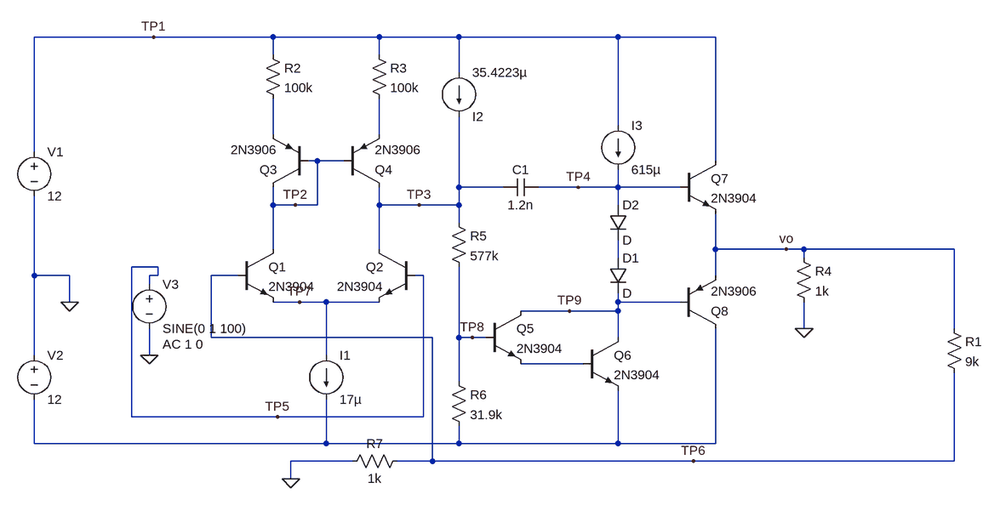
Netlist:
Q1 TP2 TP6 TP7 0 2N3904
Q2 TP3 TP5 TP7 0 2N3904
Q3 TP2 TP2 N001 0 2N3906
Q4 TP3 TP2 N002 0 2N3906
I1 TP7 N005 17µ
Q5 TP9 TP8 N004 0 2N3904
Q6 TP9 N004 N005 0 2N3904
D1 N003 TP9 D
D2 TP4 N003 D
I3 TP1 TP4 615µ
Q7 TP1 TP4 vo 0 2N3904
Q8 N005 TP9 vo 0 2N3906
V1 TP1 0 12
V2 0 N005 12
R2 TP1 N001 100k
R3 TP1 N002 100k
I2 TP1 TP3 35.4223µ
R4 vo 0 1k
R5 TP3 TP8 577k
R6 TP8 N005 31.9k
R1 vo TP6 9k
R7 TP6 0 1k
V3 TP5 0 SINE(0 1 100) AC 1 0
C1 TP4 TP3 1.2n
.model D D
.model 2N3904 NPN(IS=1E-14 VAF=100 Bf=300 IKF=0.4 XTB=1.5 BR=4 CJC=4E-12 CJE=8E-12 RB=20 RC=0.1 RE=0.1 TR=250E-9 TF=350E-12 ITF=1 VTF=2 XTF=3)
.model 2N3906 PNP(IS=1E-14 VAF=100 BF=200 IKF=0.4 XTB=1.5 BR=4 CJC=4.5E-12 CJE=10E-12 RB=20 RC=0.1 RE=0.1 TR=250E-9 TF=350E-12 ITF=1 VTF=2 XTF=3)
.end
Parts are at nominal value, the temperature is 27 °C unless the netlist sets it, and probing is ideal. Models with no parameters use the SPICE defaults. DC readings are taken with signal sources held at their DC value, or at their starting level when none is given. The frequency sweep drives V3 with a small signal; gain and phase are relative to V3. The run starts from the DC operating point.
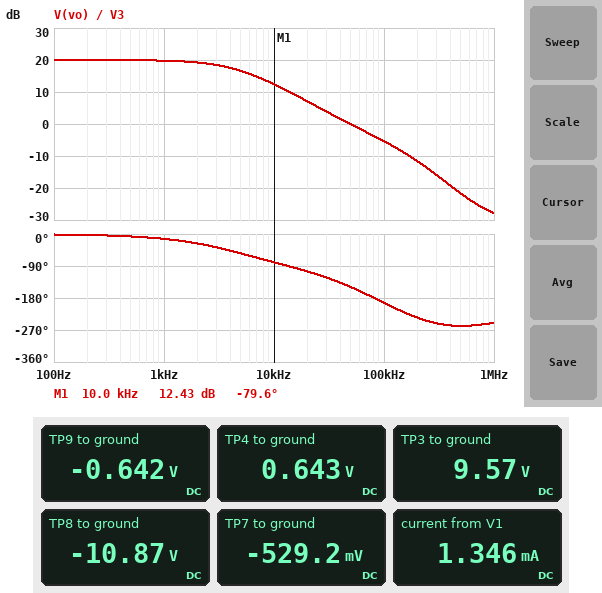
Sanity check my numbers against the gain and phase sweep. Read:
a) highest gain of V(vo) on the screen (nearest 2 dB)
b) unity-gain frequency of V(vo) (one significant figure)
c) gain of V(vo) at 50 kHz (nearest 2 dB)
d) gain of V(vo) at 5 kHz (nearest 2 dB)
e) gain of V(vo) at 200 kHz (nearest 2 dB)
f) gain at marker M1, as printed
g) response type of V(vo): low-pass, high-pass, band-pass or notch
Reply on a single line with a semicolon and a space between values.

20 dB; 50 kHz; 0 dB; 16 dB; -12 dB; 12.43 dB; low-pass
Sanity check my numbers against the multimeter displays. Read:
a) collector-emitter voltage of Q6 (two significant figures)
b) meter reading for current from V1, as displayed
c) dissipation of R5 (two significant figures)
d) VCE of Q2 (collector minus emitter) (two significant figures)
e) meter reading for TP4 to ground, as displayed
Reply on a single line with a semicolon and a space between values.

11 V; 1.346 mA; 720 µW; 10 V; 0.643 V
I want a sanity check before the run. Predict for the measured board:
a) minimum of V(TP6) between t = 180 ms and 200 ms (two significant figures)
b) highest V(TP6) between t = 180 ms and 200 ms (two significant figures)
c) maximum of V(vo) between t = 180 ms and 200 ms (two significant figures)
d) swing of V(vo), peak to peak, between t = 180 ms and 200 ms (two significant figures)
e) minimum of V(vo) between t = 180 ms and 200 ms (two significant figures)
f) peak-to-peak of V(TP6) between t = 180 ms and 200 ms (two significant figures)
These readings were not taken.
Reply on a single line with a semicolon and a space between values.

-1.0 V; 1.0 V; 10 V; 20 V; -10 V; 2.0 V
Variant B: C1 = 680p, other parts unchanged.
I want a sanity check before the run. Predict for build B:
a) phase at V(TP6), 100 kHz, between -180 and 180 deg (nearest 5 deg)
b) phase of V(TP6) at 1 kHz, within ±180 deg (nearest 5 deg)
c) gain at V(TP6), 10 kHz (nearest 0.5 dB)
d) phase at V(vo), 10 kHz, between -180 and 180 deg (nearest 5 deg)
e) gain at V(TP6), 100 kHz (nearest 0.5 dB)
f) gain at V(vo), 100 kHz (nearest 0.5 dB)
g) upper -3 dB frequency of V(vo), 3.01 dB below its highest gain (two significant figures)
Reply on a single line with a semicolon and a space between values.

165 deg; -10 deg; -4.0 dB; -60 deg; -23.0 dB; -2.5 dB; 8.5 kHz
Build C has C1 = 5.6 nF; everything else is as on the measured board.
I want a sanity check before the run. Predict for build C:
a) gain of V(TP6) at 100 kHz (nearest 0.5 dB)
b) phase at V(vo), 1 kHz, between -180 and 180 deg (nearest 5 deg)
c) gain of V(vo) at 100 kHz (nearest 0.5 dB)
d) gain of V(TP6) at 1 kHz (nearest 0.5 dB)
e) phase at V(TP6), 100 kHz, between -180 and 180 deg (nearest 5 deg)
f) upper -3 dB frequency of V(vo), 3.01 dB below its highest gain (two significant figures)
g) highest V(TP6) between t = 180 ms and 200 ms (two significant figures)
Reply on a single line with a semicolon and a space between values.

-26.5 dB; -50 deg; -8.0 dB; -3.5 dB; 120 deg; 940 Hz; 710 mV
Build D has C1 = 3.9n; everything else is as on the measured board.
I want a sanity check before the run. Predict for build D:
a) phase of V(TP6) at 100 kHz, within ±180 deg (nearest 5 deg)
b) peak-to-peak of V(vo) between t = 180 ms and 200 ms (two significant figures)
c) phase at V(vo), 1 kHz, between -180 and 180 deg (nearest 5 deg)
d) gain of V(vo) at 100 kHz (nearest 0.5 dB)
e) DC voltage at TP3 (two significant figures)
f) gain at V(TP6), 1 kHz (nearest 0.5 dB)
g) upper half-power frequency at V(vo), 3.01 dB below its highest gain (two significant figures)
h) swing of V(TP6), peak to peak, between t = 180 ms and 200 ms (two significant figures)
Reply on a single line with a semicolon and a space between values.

125 deg; 19 V; -40 deg; -8.0 dB; 9.6 V; -2.0 dB; 1.4 kHz; 1.9 V
